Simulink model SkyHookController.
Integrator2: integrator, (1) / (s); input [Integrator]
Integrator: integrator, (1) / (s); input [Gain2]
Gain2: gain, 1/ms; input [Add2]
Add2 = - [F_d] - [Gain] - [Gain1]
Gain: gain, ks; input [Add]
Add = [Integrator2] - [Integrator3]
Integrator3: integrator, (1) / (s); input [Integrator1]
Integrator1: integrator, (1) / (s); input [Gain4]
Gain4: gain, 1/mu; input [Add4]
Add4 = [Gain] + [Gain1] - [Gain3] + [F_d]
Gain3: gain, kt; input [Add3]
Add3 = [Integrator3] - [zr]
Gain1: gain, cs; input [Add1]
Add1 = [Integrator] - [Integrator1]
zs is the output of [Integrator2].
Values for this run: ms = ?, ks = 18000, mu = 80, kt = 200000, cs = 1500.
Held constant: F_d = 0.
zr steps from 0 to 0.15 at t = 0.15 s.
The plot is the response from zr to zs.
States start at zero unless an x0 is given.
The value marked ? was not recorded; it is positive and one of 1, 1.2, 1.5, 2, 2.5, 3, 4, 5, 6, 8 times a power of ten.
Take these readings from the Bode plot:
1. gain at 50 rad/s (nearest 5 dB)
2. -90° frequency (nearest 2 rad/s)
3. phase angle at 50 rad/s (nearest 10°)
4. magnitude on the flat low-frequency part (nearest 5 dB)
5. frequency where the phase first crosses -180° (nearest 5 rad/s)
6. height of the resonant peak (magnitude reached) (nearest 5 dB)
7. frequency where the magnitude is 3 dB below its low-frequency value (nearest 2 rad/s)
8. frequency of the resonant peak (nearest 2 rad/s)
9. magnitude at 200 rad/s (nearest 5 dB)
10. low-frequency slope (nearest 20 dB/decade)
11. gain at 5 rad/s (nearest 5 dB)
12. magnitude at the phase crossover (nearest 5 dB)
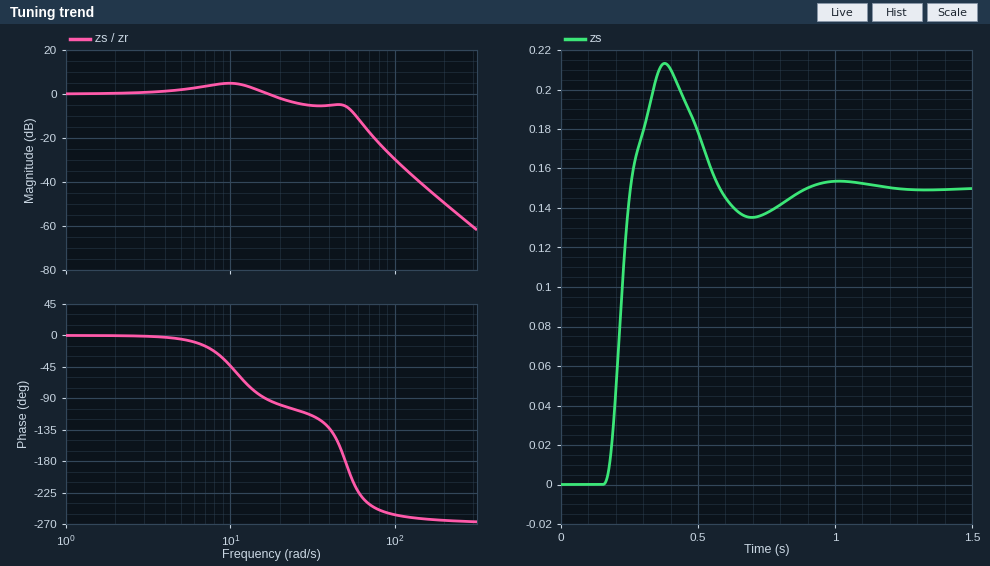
-5 dB
16 rad/s
-180°
0 dB
50 rad/s
5 dB
22 rad/s
10 rad/s
-50 dB
0 dB/decade
0 dB
-5 dB
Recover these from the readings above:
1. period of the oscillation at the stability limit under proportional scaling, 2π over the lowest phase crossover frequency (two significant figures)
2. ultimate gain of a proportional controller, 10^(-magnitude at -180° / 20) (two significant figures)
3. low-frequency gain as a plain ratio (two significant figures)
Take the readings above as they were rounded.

0.13 s
1.8
1.0
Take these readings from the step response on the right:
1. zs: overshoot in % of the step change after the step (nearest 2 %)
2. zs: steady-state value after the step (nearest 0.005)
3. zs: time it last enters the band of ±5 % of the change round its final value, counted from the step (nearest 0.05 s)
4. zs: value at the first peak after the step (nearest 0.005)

42 %
0.150
0.65 s
0.215
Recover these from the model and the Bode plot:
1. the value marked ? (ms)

150
